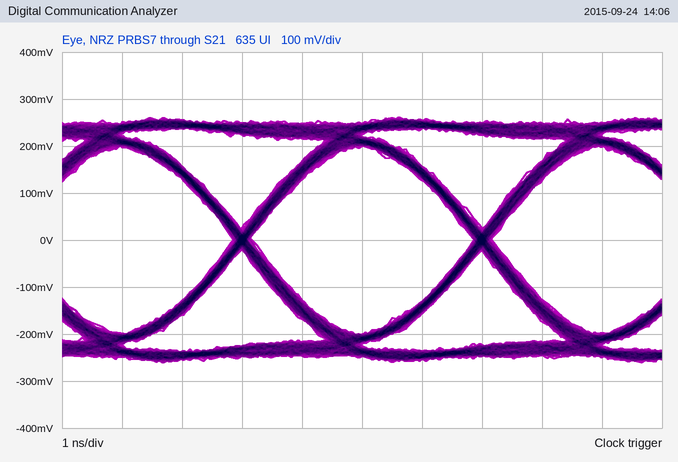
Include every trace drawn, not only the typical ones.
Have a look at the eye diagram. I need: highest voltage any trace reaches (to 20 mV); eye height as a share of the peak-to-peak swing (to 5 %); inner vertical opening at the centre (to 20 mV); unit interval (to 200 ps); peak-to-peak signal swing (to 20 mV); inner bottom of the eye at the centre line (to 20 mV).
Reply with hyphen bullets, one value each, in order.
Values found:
- 260 mV
- 75 %
- 400 mV
- 4.0 ns
- 520 mV
- -200 mV
